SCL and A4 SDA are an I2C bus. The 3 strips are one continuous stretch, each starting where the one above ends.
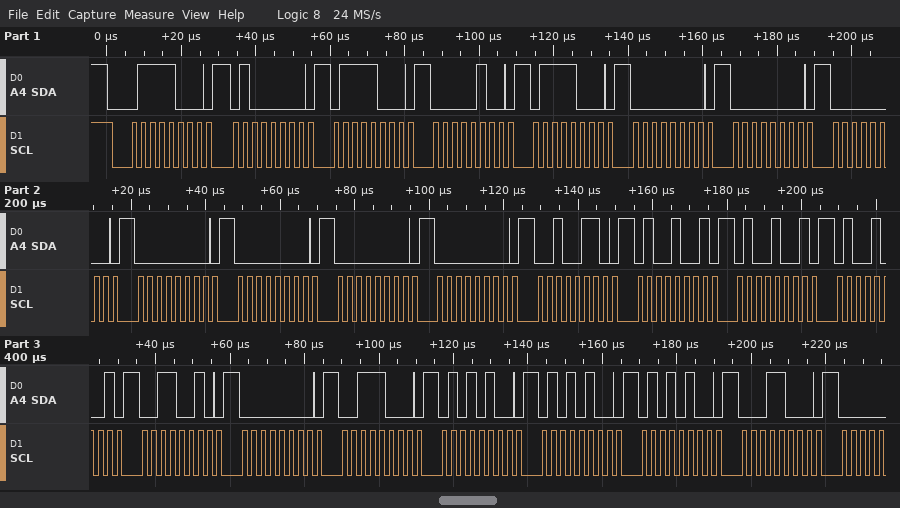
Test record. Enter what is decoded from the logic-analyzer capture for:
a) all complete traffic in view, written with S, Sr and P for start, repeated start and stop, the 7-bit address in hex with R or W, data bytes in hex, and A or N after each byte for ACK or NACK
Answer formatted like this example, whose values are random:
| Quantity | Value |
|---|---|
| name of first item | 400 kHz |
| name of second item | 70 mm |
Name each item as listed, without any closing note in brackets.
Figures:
| Quantity | Value |
|---|---|
| all complete traffic in view, written with S, Sr and P for start, repeated start and stop, the 7-bit address in hex with R or W, data bytes in hex, and A or N after each byte for ACK or NACK | S 3CW A 40 A 78 A 04 A 78 A 00 A 00 A 00 A 00 A 00 A 00 A 00 A 26 A 49 A 49 A 49 A 32 A 00 A 38 A 54 A 54 A 54 A 18 A |
